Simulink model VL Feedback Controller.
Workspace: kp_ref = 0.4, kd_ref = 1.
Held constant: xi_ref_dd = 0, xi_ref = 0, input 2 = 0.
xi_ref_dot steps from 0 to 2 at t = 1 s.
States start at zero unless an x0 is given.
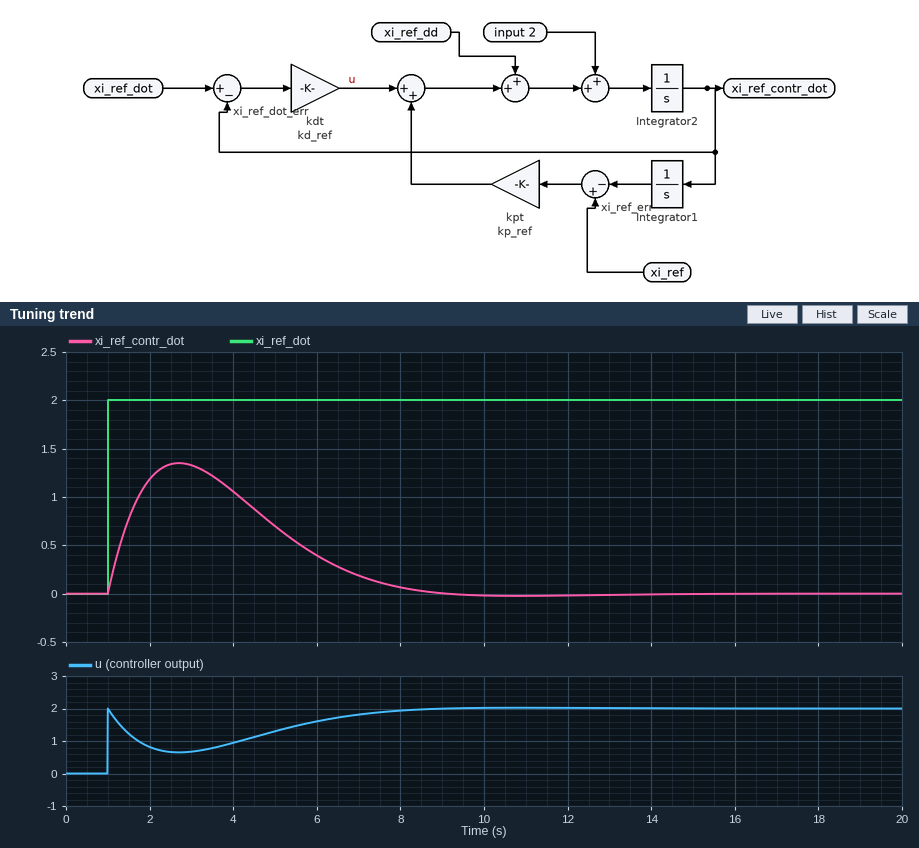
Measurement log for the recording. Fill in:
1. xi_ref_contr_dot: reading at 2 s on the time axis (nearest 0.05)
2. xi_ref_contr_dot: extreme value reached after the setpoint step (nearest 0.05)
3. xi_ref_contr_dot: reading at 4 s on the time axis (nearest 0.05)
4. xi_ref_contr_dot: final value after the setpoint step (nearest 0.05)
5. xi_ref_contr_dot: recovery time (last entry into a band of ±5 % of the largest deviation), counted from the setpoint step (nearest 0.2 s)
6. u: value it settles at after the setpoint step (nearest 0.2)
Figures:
1.20
1.35
1.05
0.00
7.0 s
2.0
